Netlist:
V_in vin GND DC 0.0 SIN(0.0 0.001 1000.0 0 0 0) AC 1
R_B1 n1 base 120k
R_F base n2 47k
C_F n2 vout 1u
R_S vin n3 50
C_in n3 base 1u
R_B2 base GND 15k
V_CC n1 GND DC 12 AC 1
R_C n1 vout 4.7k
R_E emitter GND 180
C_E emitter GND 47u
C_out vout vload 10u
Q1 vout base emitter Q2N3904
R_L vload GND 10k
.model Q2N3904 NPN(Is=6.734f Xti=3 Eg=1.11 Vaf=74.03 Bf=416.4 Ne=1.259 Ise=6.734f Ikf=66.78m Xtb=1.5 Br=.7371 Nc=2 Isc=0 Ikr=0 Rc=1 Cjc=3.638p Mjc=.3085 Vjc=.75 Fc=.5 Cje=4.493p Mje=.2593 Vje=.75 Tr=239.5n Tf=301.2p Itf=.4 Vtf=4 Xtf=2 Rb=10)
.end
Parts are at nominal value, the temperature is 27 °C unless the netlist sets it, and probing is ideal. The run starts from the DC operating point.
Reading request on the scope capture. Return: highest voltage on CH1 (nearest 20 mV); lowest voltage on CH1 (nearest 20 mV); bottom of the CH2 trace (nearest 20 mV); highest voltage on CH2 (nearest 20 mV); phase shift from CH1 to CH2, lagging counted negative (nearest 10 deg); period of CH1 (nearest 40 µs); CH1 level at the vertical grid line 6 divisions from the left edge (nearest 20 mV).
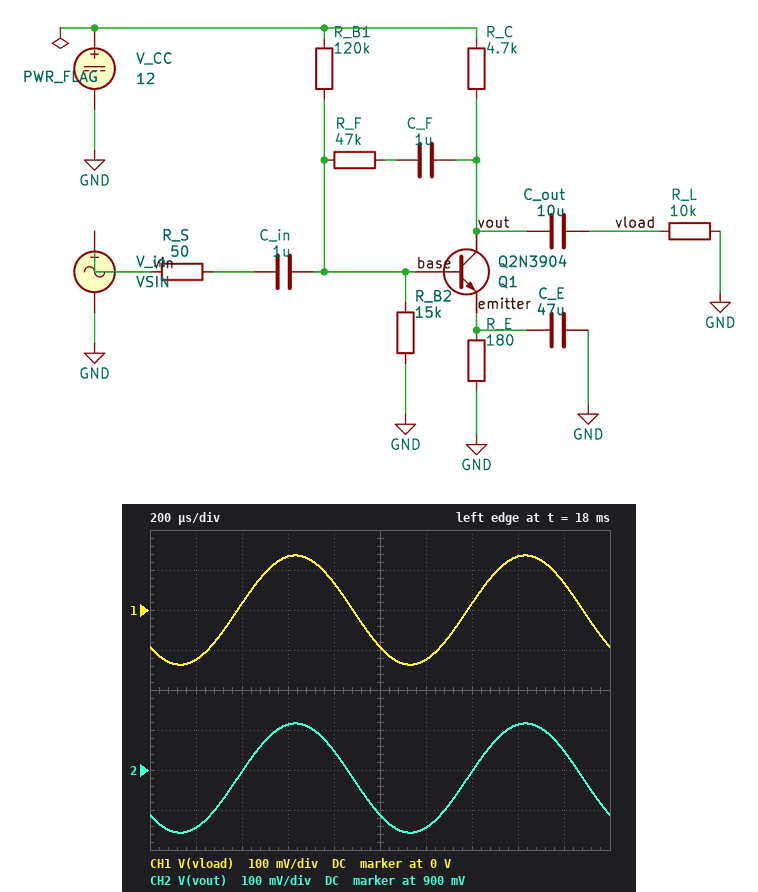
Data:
140 mV
-140 mV
740 mV
1.02 V
0 deg
1.00 ms
-120 mV
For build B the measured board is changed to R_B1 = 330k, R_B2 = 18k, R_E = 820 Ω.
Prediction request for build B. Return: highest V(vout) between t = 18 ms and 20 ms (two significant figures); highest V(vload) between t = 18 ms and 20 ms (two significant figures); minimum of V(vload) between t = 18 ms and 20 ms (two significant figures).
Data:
12 V
4.6 mV
-4.7 mV
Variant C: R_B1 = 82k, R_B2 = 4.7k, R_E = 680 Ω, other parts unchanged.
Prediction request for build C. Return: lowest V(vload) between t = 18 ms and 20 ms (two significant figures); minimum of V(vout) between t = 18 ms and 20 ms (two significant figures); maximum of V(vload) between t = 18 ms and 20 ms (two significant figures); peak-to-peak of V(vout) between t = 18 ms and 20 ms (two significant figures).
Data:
-8.6 mV
12 V
8.4 mV
17 mV
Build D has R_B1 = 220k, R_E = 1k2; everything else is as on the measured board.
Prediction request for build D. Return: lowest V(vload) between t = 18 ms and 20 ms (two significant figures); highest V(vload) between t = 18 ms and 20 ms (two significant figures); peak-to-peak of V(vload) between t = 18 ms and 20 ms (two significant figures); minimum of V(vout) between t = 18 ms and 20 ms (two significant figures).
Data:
-13 mV
13 mV
27 mV
11 V
